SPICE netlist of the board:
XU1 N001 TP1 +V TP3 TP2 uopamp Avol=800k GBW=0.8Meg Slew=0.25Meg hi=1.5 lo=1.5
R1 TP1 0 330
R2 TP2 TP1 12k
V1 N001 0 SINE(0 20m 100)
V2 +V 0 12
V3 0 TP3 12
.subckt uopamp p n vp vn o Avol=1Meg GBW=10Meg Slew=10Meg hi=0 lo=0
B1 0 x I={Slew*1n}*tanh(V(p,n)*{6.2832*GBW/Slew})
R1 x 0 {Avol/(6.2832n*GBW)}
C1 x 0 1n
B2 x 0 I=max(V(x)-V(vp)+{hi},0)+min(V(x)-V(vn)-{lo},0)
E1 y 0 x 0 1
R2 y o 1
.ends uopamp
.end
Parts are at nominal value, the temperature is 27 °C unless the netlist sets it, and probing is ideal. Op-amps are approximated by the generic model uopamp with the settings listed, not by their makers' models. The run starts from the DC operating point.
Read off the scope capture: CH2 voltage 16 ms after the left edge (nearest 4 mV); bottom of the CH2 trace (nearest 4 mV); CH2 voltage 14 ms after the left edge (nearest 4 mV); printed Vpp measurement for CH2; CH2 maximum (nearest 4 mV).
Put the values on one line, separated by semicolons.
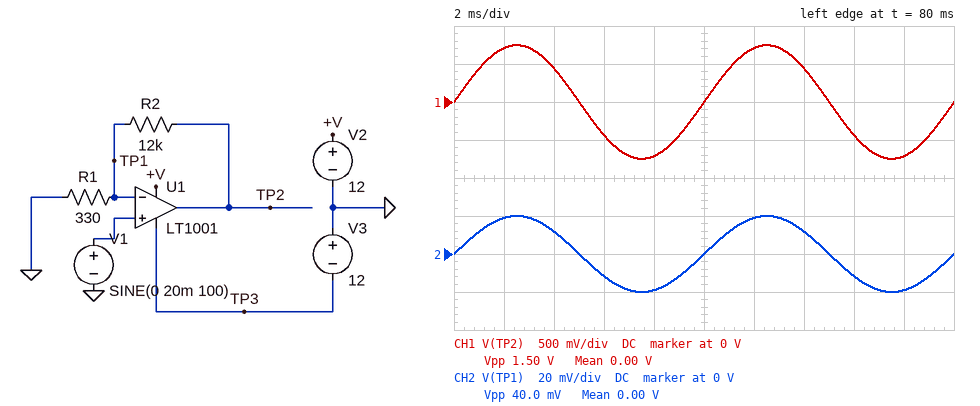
-12 mV; -20 mV; 12 mV; 40.0 mV; 20 mV
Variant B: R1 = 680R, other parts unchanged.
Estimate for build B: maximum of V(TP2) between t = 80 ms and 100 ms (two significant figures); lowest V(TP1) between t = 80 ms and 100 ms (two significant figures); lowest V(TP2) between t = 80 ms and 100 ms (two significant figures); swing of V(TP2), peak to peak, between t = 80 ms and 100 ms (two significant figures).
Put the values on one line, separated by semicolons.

370 mV; -20 mV; -370 mV; 750 mV
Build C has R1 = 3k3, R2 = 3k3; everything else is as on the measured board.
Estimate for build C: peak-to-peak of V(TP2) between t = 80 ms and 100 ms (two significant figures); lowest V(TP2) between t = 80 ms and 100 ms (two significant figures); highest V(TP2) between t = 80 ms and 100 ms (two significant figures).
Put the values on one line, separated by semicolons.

80 mV; -40 mV; 40 mV
